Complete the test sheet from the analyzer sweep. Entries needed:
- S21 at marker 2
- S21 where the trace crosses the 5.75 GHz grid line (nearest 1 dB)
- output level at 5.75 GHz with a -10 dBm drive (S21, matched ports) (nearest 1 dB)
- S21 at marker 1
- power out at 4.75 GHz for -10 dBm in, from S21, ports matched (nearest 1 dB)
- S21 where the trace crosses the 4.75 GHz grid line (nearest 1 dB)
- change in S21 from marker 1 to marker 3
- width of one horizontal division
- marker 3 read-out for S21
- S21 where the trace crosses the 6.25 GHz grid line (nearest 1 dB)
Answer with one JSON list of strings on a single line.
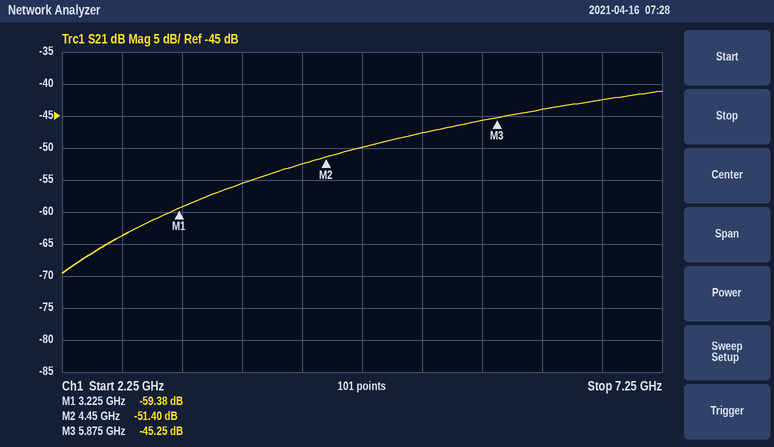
["-51.40 dB", "-46 dB", "-56 dBm", "-59.38 dB", "-60 dBm", "-50 dB", "14.13 dB", "500 MHz", "-45.25 dB", "-44 dB"]
